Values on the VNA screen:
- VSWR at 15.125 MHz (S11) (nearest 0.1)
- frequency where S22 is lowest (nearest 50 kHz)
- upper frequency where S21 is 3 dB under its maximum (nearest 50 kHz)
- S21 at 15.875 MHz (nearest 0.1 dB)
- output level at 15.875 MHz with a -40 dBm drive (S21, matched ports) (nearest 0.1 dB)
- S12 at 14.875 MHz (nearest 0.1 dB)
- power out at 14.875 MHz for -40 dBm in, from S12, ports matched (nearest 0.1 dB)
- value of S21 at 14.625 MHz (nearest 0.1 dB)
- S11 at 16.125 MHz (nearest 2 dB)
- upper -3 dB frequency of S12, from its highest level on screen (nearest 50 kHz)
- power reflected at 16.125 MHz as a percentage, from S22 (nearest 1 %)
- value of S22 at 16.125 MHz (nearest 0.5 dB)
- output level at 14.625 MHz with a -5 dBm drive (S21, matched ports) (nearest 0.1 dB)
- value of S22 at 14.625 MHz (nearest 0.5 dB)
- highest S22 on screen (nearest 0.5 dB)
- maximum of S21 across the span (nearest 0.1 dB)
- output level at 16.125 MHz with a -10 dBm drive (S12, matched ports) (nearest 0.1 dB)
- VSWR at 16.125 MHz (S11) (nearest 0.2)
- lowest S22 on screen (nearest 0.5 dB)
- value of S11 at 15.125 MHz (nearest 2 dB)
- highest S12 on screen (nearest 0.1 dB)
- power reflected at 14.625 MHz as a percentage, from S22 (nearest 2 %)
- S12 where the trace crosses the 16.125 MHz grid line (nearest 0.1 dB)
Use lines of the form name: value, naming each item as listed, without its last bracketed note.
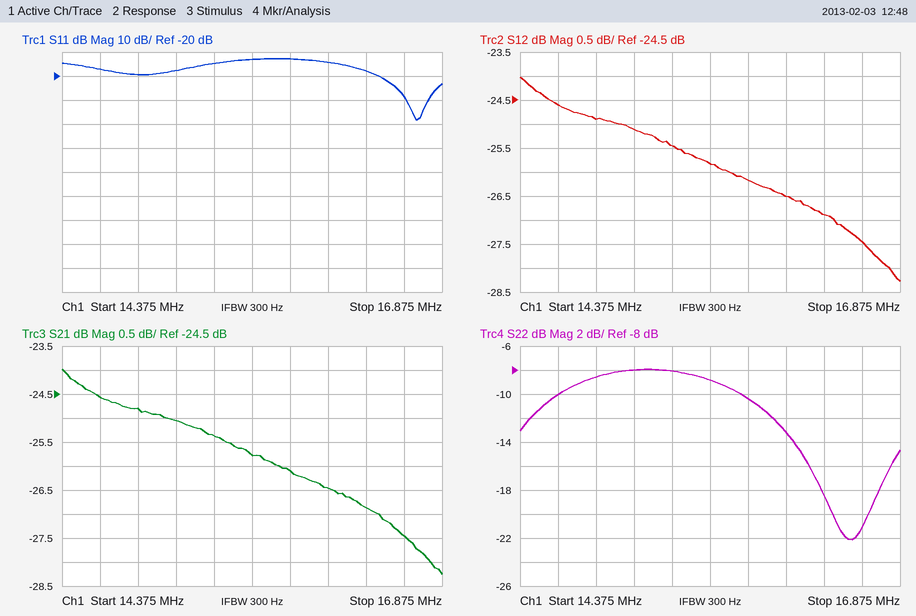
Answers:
VSWR at 15.125 MHz (S11): 1.3
frequency where S22 is lowest: 16.55 MHz
upper frequency where S21 is 3 dB under its maximum: 16.45 MHz
S21 at 15.875 MHz: -26.1 dB
output level at 15.875 MHz with a -40 dBm drive (S21, matched ports): -66.1 dBm
S12 at 14.875 MHz: -24.9 dB
power out at 14.875 MHz for -40 dBm in, from S12, ports matched: -64.9 dBm
value of S21 at 14.625 MHz: -24.6 dB
S11 at 16.125 MHz: -14 dB
upper -3 dB frequency of S12, from its highest level on screen: 16.45 MHz
power reflected at 16.125 MHz as a percentage, from S22: 5 %
value of S22 at 16.125 MHz: -13.0 dB
output level at 14.625 MHz with a -5 dBm drive (S21, matched ports): -29.6 dBm
value of S22 at 14.625 MHz: -10.0 dB
highest S22 on screen: -8.0 dB
maximum of S21 across the span: -24.0 dB
output level at 16.125 MHz with a -10 dBm drive (S12, matched ports): -36.5 dBm
VSWR at 16.125 MHz (S11): 1.4
lowest S22 on screen: -22.0 dB
value of S11 at 15.125 MHz: -18 dB
highest S12 on screen: -24.0 dB
power reflected at 14.625 MHz as a percentage, from S22: 10 %
S12 where the trace crosses the 16.125 MHz grid line: -26.5 dB
